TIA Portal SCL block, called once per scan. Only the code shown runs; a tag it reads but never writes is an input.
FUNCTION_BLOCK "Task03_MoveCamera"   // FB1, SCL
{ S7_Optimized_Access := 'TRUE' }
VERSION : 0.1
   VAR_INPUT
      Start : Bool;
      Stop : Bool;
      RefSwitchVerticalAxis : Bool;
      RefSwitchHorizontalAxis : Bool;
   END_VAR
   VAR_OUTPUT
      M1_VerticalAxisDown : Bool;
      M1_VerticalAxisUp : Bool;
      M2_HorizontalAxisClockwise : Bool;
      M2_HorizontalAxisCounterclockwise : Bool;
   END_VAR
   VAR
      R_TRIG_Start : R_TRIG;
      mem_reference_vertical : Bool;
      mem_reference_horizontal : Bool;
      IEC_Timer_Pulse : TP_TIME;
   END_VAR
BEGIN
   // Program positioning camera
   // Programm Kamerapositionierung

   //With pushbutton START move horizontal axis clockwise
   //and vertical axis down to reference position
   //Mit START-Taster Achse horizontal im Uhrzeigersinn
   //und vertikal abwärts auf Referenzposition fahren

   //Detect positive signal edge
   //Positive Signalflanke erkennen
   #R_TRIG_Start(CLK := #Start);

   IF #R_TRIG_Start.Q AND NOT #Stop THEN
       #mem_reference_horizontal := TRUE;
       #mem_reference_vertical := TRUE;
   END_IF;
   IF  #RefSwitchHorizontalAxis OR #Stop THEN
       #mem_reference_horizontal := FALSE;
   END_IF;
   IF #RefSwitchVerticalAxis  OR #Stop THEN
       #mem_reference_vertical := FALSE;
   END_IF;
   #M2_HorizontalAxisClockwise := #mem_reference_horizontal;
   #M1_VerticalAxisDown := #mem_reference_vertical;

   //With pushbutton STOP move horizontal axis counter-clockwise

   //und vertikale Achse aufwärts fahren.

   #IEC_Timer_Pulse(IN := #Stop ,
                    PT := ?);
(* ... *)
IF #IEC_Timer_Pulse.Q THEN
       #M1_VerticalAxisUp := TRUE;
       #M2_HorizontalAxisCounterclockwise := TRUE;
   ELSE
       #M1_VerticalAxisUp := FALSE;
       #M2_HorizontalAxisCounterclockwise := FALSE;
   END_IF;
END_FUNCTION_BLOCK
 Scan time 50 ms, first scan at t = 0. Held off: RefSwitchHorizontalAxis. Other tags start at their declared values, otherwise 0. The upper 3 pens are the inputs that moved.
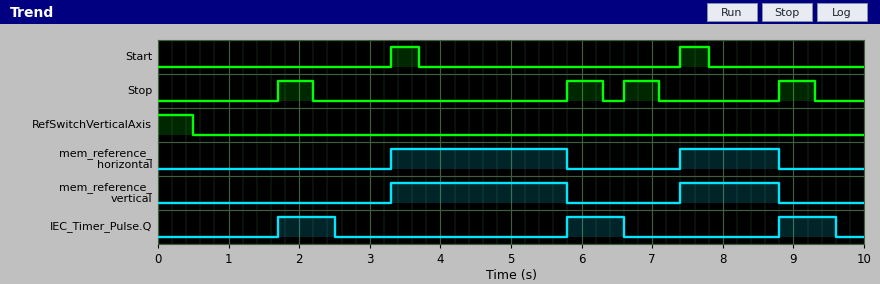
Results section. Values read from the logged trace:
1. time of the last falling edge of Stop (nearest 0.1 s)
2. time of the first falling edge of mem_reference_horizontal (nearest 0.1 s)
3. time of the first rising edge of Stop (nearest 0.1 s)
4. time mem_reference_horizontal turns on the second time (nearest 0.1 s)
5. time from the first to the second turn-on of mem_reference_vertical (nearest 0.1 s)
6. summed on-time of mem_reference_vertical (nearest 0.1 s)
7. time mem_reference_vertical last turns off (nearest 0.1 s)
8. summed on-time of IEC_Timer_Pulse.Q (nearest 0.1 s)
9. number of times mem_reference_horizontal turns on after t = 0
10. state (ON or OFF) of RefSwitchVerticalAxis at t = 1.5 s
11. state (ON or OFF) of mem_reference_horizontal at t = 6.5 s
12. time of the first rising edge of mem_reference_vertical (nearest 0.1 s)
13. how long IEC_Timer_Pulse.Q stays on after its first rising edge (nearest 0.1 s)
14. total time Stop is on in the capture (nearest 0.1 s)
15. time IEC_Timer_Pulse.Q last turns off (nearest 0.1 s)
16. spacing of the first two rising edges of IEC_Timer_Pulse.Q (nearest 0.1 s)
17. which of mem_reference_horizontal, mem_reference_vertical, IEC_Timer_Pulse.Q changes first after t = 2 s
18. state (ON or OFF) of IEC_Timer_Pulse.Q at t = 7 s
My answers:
9.3 s
5.8 s
1.7 s
7.4 s
4.1 s
3.9 s
8.8 s
2.4 s
2
OFF
OFF
3.3 s
0.8 s
2.0 s
9.6 s
4.1 s
IEC_Timer_Pulse.Q
OFF
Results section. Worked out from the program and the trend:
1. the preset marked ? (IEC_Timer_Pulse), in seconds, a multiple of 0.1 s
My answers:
0.8 s
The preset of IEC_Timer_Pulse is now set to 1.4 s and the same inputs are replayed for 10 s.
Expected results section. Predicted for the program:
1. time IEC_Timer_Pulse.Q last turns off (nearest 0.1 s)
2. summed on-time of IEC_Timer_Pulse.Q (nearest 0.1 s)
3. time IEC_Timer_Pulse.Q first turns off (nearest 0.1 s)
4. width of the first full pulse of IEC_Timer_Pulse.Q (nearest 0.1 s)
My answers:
7.2 s
4.0 s
3.1 s
1.4 s
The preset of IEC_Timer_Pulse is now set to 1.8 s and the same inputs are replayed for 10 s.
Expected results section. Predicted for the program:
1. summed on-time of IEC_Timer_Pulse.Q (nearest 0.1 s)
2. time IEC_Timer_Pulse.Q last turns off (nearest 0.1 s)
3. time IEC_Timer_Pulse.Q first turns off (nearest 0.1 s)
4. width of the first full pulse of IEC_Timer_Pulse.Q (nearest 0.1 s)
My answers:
4.8 s
7.6 s
3.5 s
1.8 s
